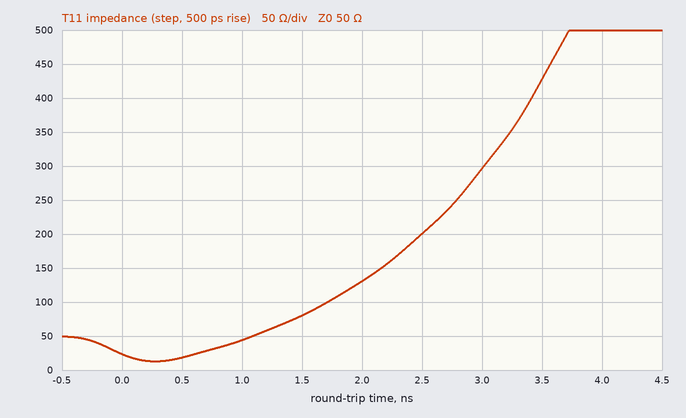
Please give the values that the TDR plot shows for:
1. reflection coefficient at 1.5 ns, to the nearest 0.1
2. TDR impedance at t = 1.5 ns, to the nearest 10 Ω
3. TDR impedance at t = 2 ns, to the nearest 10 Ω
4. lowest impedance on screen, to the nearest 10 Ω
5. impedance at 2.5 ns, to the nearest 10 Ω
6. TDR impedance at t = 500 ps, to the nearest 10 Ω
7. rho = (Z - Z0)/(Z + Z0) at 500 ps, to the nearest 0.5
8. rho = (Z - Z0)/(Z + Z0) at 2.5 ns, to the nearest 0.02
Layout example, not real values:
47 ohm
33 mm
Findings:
+0.2
80 Ω
130 Ω
10 Ω
200 Ω
20 Ω
-0.5
+0.60
